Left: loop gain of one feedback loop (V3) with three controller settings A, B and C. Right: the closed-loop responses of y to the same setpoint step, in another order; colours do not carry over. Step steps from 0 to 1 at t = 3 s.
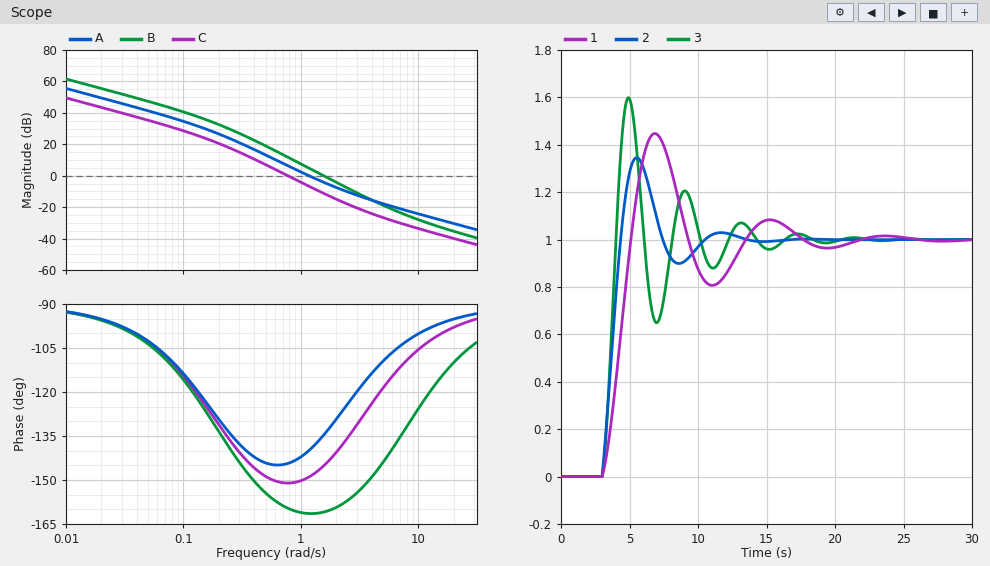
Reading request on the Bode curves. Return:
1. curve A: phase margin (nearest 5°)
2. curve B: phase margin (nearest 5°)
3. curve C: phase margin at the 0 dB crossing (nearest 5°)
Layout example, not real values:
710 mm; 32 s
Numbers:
40°; 20°; 30°
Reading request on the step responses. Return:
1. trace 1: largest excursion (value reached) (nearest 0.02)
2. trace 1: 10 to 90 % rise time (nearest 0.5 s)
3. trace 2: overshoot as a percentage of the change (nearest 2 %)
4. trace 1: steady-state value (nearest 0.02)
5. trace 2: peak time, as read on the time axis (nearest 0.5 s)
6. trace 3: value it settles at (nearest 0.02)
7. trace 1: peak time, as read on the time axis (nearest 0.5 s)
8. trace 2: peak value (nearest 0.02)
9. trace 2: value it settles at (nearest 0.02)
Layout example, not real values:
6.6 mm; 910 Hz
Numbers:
1.44; 1.5 s; 34 %; 1.00; 5.5 s; 1.00; 7.0 s; 1.34; 1.00
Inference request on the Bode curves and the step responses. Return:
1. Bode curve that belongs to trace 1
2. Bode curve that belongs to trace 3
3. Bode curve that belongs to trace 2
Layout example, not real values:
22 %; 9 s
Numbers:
C; B; A
